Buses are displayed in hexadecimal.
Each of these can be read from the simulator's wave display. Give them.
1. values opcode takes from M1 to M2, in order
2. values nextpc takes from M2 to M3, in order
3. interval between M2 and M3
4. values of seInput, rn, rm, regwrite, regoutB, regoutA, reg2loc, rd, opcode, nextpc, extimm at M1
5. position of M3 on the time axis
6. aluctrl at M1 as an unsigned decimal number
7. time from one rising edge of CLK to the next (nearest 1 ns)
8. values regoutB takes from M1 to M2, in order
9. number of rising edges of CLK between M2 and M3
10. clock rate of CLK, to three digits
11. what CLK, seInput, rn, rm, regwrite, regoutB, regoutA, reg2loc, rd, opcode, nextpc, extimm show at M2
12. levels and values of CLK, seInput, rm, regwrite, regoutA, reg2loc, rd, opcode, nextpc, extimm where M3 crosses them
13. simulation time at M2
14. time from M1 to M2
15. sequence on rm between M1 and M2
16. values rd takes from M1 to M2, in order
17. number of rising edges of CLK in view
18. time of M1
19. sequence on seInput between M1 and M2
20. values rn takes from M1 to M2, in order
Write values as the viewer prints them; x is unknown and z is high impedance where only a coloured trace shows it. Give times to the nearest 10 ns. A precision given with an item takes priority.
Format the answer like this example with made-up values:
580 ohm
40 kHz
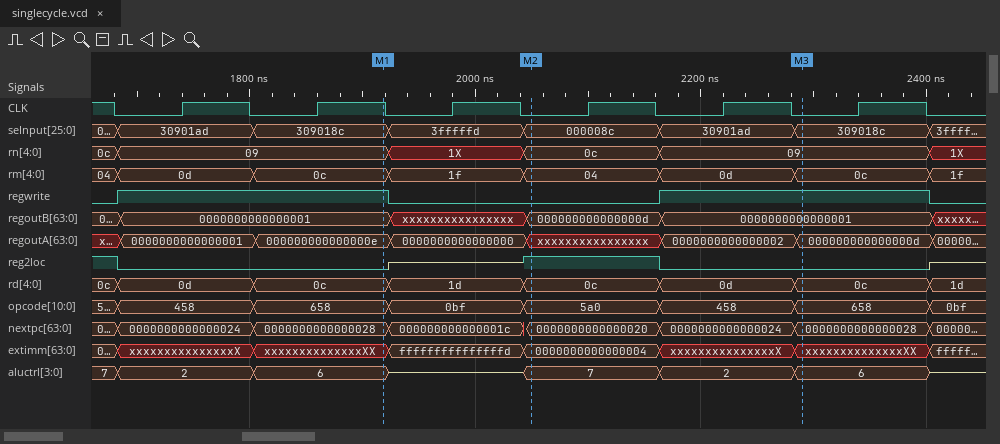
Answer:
658, 0bf, 5a0
0000000000000020, 0000000000000024, 0000000000000028
240 ns
seInput=309018c, rn=09, rm=0c, regwrite=1, regoutB=0000000000000001, regoutA=000000000000000e, reg2loc=0, rd=0c, opcode=658, nextpc=0000000000000028, extimm=xxxxxxxxxxxxxxXX
2290 ns
6
120 ns
0000000000000001, xxxxxxxxxxxxxxxx, 000000000000000d
2
8.33 MHz
CLK=0, seInput=000008c, rn=0c, rm=04, regwrite=0, regoutB=000000000000000d, regoutA=xxxxxxxxxxxxxxxx, reg2loc=1, rd=0c, opcode=5a0, nextpc=0000000000000020, extimm=0000000000000004
CLK=0, seInput=309018c, rm=0c, regwrite=1, regoutA=000000000000000d, reg2loc=0, rd=0c, opcode=658, nextpc=0000000000000028, extimm=xxxxxxxxxxxxxxXX
2050 ns
130 ns
0c, 1f, 04
0c, 1d, 0c
6
1920 ns
309018c, 3fffffd, 000008c
09, 1X, 0c
